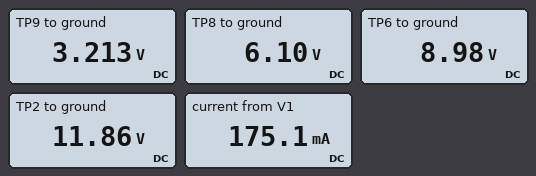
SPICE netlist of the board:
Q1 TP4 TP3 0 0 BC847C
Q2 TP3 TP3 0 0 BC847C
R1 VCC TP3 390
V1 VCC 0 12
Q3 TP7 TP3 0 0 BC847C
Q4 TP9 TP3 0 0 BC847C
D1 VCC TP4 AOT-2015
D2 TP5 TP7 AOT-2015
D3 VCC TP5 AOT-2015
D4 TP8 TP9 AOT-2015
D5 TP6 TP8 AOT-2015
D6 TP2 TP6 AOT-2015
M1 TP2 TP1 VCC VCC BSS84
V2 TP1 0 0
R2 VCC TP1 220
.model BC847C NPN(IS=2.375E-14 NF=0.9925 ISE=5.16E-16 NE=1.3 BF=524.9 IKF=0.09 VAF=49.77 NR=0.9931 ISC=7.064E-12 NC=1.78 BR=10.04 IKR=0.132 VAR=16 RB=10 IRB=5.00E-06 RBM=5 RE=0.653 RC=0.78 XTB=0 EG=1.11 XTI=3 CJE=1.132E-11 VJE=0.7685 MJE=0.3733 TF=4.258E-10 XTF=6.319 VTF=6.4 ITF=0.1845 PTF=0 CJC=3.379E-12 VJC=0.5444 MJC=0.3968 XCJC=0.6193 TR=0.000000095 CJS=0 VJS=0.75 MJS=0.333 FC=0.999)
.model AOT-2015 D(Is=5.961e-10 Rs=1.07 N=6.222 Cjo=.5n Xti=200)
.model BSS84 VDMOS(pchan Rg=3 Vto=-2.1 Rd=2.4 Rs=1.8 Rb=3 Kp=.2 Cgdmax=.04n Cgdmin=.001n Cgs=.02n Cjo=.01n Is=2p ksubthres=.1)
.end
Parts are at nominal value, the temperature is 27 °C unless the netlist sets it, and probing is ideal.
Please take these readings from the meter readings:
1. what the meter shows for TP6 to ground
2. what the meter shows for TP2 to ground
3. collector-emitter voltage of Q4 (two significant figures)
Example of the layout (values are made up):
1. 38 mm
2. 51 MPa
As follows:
1. 8.98 V
2. 11.86 V
3. 3.2 V
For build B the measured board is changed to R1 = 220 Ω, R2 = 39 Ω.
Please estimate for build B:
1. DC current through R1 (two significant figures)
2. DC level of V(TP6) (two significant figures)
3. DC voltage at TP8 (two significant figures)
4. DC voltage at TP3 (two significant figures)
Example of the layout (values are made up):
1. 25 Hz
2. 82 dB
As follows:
1. 51 mA
2. 8.8 V
3. 5.8 V
4. 780 mV
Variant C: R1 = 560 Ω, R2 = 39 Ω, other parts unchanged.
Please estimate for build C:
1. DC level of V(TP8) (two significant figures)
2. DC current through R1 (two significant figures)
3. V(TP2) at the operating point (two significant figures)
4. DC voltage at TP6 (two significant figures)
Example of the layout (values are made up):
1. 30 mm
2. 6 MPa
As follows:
1. 6.3 V
2. 20 mA
3. 12 V
4. 9.1 V
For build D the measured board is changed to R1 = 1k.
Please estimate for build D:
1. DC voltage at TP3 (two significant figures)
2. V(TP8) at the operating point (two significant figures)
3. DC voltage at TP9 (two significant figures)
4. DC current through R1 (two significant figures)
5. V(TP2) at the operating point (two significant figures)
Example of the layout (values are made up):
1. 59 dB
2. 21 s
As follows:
1. 700 mV
2. 6.5 V
3. 3.8 V
4. 11 mA
5. 12 V
